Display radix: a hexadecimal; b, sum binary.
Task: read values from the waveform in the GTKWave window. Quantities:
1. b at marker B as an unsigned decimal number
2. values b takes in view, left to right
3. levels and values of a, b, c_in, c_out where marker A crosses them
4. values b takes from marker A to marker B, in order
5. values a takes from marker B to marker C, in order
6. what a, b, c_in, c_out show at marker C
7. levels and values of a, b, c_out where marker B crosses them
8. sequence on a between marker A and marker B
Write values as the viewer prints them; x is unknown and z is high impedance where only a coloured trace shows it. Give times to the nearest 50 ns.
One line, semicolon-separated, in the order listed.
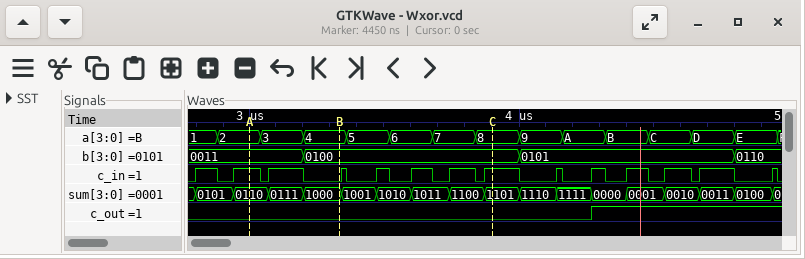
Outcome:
4; 0011, 0100, 0101, 0110; a=2, b=0011, c_in=1, c_out=0; 0011, 0100; 4, 5, 6, 7, 8; a=8, b=0100, c_in=1, c_out=0; a=4, b=0100, c_out=0; 2, 3, 4
